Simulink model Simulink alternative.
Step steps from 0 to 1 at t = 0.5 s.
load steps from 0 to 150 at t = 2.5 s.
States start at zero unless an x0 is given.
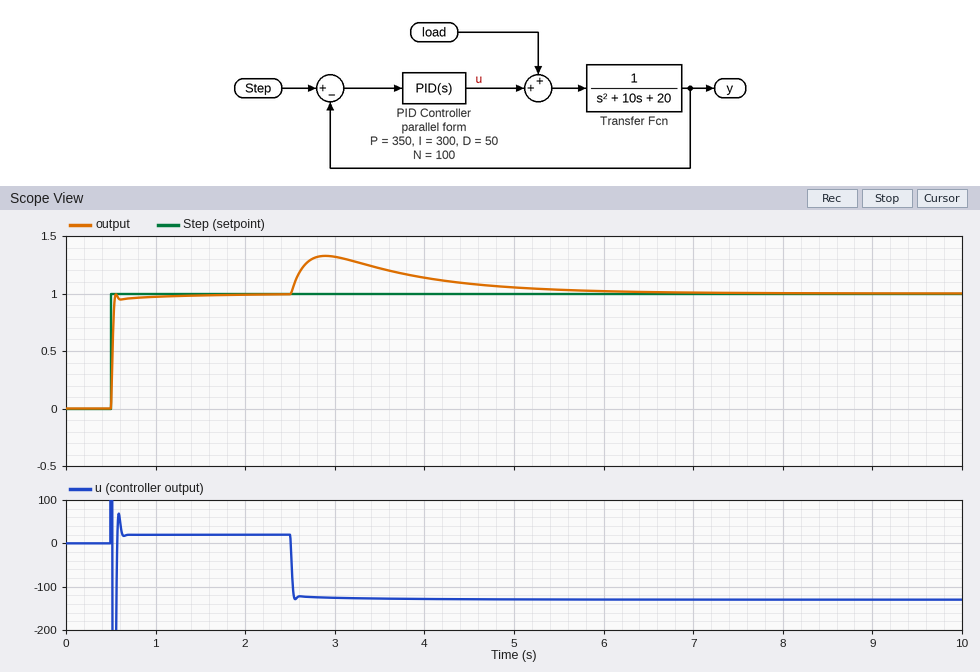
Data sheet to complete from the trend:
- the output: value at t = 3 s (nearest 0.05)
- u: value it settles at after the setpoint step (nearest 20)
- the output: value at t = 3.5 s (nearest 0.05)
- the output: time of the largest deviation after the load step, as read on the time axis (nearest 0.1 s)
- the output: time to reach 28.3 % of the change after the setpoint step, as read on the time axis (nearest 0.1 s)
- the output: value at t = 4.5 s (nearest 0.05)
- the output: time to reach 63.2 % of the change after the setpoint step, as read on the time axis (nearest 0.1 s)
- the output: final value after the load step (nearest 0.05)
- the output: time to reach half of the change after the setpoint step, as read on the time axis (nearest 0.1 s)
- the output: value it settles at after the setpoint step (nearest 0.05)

1.30
20
1.20
2.9 s
0.5 s
1.10
0.5 s
1.00
0.5 s
1.00
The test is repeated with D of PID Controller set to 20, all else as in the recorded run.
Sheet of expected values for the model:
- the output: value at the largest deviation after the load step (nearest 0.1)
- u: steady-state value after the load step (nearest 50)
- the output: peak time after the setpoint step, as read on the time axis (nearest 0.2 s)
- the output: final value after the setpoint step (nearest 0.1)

1.4
-150
0.6 s
1.0
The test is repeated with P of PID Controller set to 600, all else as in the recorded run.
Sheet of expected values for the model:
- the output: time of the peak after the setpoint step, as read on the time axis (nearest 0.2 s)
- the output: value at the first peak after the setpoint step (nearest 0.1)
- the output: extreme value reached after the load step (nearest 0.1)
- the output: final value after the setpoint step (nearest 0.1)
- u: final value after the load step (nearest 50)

0.6 s
1.1
1.2
1.0
-150
